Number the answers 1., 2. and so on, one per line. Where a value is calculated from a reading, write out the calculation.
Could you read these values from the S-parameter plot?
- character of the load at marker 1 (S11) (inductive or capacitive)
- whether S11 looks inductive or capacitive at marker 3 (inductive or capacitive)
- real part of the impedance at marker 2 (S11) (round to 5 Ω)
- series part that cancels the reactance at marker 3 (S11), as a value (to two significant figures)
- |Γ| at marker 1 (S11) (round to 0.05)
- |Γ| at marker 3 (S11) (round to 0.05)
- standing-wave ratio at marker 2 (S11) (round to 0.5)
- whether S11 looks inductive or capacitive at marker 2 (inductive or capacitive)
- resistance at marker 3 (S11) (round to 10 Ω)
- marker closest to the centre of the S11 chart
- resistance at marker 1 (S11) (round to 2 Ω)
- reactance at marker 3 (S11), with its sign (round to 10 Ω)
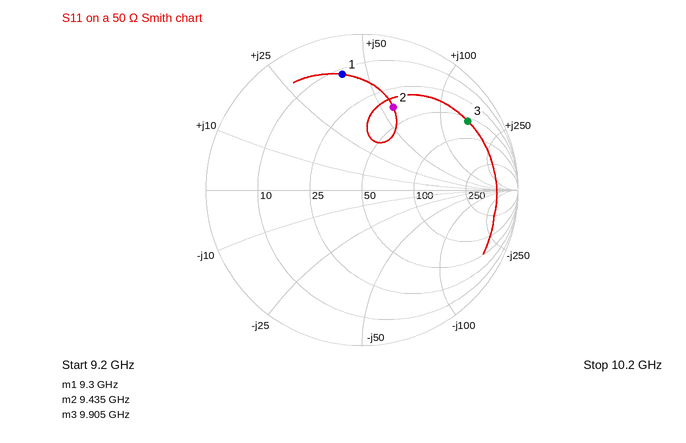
1. inductive
2. inductive
3. 35 Ω
4. C = 1/(2π × 9.905 GHz × 150 Ω) ≈ 107 fF, so 110 fF to two significant figures
5. 0.75
6. 0.80
7. 3.5
8. inductive
9. 60 Ω
10. marker 2
11. 12 Ω
12. +150 Ω
